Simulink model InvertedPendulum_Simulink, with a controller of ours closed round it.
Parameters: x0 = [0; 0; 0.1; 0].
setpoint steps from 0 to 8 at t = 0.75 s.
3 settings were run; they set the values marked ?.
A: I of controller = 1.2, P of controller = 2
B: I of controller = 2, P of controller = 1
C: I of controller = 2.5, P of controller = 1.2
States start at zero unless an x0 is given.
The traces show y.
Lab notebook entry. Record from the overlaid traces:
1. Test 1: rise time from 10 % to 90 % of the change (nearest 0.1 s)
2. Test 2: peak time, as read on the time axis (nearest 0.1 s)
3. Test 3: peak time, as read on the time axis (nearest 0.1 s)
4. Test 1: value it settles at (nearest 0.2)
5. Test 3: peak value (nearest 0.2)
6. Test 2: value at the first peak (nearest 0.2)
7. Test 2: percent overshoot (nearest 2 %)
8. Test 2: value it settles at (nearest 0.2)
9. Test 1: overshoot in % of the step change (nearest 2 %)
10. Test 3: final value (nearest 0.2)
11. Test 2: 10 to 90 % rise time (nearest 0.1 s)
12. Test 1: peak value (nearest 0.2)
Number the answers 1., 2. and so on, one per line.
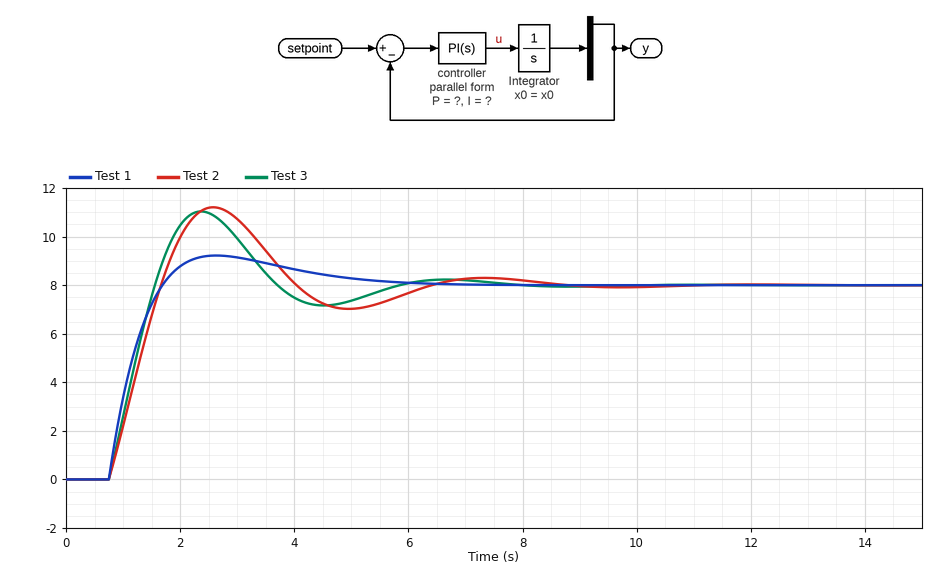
1. 0.7 s
2. 2.6 s
3. 2.4 s
4. 8.0
5. 11.0
6. 11.2
7. 40 %
8. 8.0
9. 16 %
10. 8.0
11. 0.7 s
12. 9.2
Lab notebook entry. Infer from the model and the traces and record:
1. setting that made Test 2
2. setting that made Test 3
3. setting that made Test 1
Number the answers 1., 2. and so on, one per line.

1. B
2. C
3. A
